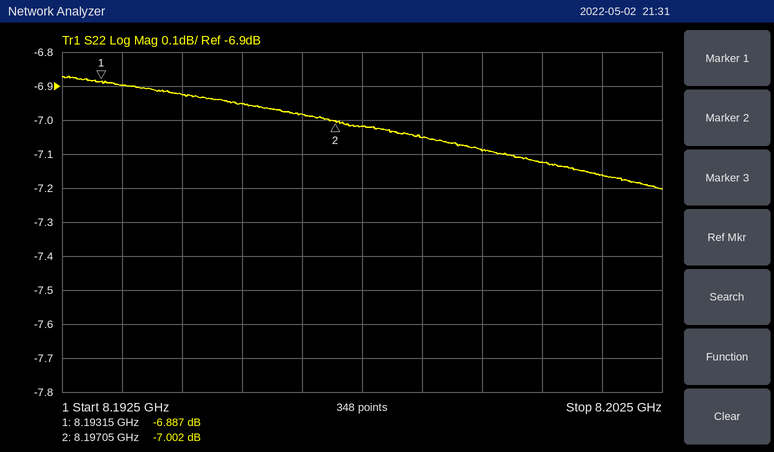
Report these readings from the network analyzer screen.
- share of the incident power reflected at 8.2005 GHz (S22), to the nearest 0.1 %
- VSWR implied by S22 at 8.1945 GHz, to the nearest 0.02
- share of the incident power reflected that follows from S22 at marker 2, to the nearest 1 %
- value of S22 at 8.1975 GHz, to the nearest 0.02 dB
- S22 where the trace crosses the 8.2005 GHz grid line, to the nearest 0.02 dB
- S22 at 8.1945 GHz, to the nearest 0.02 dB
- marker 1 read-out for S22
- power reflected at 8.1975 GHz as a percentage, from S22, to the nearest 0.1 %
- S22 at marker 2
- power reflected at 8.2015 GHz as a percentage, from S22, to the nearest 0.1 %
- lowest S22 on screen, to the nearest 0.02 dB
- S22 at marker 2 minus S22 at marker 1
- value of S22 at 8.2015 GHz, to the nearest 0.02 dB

19.4 %
2.64
20 %
-7.02 dB
-7.12 dB
-6.92 dB
-6.887 dB
19.9 %
-7.002 dB
19.2 %
-7.20 dB
-0.115 dB
-7.16 dB
